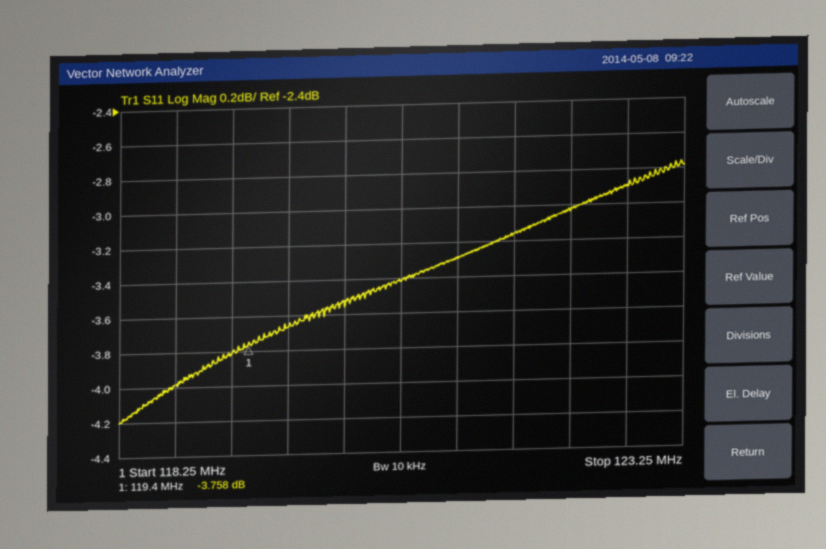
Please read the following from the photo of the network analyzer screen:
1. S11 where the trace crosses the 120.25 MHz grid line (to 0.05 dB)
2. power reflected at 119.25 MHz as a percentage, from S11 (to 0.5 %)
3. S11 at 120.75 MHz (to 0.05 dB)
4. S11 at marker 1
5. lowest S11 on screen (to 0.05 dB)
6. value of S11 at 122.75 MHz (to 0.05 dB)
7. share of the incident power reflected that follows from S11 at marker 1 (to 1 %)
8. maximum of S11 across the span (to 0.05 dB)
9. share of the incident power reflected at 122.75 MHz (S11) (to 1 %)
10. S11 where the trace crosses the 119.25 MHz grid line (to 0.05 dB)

-3.55 dB
41.5 %
-3.40 dB
-3.758 dB
-4.20 dB
-2.90 dB
42 %
-2.75 dB
51 %
-3.80 dB
